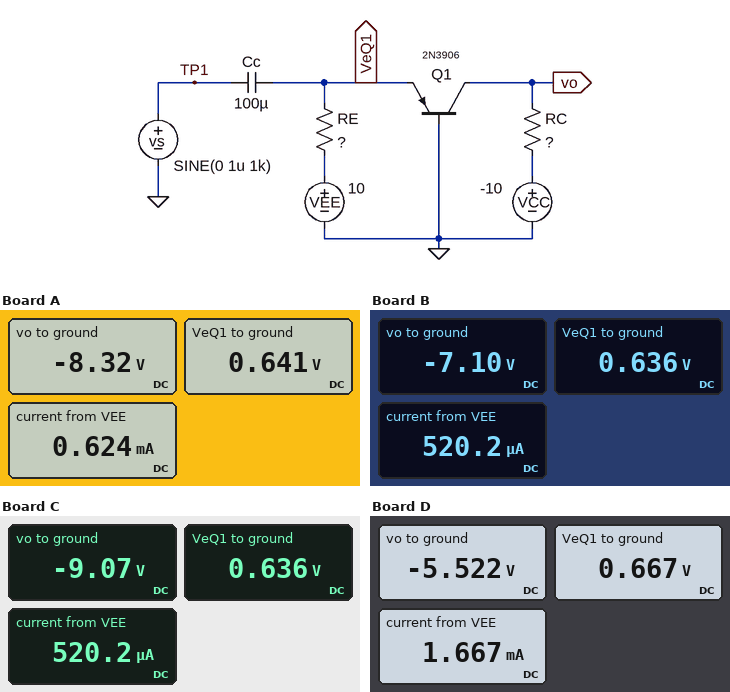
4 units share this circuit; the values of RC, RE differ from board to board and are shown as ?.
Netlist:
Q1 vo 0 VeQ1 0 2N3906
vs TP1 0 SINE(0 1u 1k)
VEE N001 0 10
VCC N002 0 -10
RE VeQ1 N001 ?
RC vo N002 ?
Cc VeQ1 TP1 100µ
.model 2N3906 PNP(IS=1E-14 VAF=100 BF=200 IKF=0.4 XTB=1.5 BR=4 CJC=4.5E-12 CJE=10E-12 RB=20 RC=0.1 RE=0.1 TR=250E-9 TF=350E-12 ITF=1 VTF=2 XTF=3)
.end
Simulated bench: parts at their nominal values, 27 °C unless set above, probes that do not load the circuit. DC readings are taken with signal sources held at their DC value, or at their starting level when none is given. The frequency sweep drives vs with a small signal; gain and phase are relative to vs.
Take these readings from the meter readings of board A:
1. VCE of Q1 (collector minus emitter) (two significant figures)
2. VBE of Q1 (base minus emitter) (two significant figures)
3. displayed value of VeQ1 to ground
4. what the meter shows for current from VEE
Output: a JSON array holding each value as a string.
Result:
["-9.0 V", "-640 mV", "0.641 V", "0.624 mA"]
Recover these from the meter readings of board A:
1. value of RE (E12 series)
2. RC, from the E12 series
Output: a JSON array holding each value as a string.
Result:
["15 kΩ", "2.7 kΩ"]
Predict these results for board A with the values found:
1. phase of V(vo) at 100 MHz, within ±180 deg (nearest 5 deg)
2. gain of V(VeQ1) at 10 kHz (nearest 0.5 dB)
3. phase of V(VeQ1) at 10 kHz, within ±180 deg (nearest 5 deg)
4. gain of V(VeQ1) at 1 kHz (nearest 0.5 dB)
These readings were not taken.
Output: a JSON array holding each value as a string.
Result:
["-90 deg", "0 dB", "0 deg", "0 dB"]
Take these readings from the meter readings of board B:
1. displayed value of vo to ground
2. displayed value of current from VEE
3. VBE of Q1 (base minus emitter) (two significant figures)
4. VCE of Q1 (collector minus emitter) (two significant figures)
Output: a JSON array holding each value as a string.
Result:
["-7.10 V", "520.2 µA", "-640 mV", "-7.7 V"]
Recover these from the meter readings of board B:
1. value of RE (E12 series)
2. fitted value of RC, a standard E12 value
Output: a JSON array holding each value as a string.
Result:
["18 kΩ", "5.6 kΩ"]
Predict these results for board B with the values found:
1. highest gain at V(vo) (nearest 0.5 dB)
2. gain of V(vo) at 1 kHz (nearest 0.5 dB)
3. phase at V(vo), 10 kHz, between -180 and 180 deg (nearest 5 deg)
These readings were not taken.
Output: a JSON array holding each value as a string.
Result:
["40.5 dB", "40.5 dB", "0 deg"]
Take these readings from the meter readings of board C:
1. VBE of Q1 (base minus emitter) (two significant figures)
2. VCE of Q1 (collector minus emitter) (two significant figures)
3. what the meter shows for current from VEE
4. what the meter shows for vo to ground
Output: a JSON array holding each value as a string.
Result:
["-640 mV", "-9.7 V", "520.2 µA", "-9.07 V"]
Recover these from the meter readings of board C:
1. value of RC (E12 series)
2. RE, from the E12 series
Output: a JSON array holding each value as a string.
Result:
["1.8 kΩ", "18 kΩ"]
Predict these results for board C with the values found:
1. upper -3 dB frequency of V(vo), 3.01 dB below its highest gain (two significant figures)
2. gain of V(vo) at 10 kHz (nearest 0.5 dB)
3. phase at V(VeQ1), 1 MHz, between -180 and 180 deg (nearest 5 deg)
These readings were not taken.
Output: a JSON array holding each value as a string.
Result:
["32 MHz", "31.0 dB", "0 deg"]
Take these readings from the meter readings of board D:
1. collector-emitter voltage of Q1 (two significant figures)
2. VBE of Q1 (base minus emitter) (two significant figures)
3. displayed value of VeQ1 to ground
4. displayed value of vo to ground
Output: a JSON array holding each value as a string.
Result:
["-6.2 V", "-670 mV", "0.667 V", "-5.522 V"]
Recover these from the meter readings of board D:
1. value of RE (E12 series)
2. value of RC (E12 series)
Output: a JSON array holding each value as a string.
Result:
["5.6 kΩ", "2.7 kΩ"]
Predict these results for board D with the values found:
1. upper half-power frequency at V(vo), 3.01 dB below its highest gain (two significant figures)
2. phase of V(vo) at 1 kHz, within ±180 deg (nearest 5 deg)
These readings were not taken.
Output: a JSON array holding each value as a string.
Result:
["12 MHz", "5 deg"]
